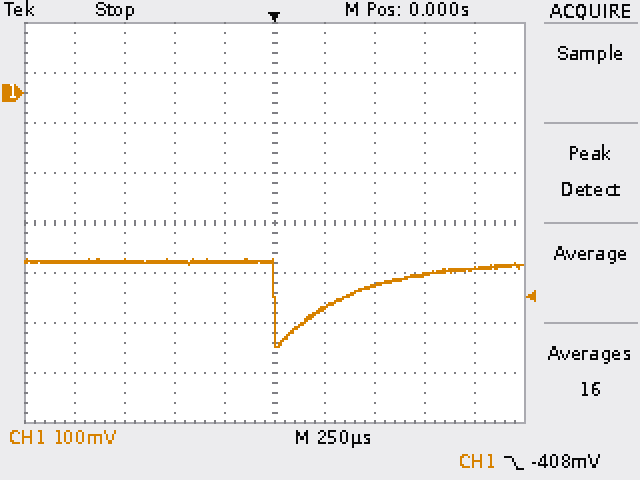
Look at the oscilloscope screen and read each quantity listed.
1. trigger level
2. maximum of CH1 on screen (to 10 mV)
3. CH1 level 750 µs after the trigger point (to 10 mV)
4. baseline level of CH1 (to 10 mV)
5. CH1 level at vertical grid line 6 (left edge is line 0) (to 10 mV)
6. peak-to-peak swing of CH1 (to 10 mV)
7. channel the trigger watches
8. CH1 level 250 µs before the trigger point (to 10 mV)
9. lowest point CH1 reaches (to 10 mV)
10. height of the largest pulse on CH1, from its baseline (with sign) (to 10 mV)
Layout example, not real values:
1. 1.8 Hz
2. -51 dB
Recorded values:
1. -408 mV
2. -330 mV
3. -360 mV
4. -340 mV
5. -430 mV
6. 180 mV
7. CH1
8. -340 mV
9. -510 mV
10. -170 mV
